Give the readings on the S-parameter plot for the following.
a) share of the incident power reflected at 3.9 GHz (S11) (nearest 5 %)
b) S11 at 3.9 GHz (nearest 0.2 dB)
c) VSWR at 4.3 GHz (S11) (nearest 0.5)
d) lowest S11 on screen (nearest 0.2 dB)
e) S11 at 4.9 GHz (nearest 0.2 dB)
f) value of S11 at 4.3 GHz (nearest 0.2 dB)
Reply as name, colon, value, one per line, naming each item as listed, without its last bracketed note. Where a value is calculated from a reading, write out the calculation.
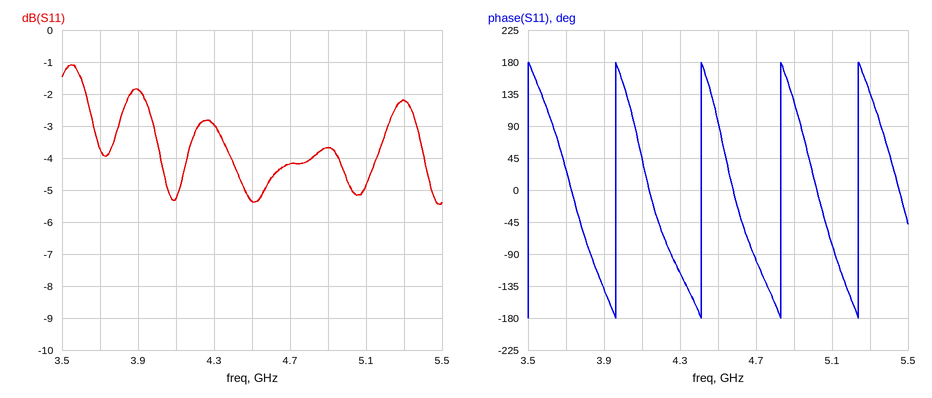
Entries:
share of the incident power reflected at 3.9 GHz (S11): 10^(-1.8/10) ≈ 66.1 %, so 65 % to the nearest 5 %
S11 at 3.9 GHz: -1.8 dB
VSWR at 4.3 GHz (S11): |Γ| = 10^(-3/20) = 0.7079; VSWR = (1 + 0.7079)/(1 − 0.7079) ≈ 5.85, so 6.0 to the nearest 0.5
lowest S11 on screen: -5.4 dB
S11 at 4.9 GHz: -3.6 dB
value of S11 at 4.3 GHz: -3.0 dB
